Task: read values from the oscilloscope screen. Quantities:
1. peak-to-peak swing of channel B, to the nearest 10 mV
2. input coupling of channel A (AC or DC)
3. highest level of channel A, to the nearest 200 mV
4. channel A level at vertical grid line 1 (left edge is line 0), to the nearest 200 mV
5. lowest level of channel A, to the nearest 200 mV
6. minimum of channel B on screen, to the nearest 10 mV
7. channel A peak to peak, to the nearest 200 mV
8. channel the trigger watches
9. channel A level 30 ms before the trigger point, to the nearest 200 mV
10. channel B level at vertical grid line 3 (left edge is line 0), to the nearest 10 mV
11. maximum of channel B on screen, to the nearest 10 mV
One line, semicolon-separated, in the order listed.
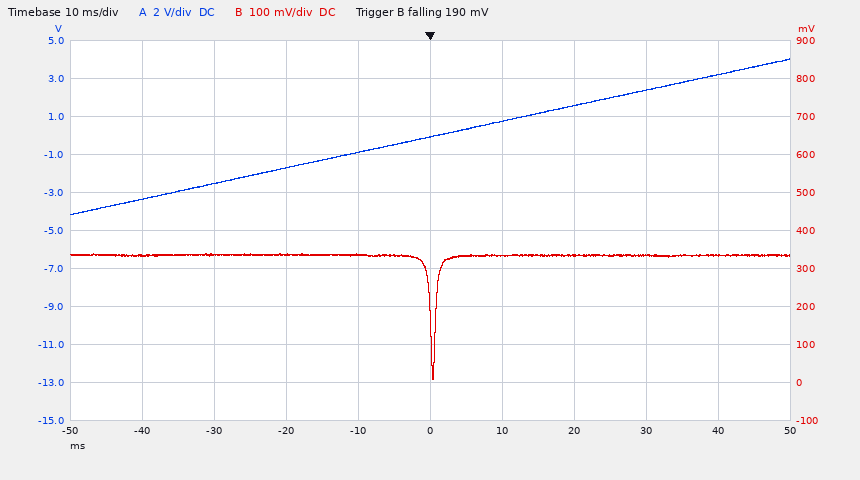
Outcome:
330 mV; DC; 4.0 V; -3.4 V; -4.2 V; 10 mV; 8.2 V; channel B; -2.6 V; 340 mV; 340 mV
